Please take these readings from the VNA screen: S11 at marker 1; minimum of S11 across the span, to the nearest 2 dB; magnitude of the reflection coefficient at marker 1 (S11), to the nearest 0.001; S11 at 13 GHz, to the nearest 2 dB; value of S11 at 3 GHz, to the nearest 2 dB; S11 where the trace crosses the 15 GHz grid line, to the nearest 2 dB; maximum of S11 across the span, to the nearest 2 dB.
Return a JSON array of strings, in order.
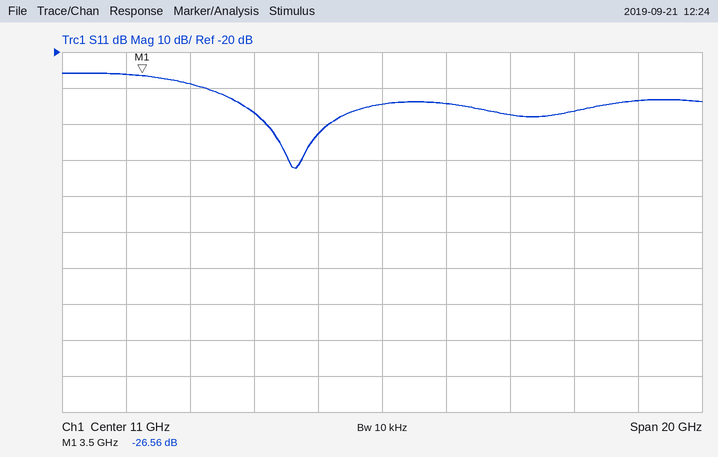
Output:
["-26.56 dB", "-52 dB", "0.047", "-34 dB", "-26 dB", "-38 dB", "-26 dB"]
